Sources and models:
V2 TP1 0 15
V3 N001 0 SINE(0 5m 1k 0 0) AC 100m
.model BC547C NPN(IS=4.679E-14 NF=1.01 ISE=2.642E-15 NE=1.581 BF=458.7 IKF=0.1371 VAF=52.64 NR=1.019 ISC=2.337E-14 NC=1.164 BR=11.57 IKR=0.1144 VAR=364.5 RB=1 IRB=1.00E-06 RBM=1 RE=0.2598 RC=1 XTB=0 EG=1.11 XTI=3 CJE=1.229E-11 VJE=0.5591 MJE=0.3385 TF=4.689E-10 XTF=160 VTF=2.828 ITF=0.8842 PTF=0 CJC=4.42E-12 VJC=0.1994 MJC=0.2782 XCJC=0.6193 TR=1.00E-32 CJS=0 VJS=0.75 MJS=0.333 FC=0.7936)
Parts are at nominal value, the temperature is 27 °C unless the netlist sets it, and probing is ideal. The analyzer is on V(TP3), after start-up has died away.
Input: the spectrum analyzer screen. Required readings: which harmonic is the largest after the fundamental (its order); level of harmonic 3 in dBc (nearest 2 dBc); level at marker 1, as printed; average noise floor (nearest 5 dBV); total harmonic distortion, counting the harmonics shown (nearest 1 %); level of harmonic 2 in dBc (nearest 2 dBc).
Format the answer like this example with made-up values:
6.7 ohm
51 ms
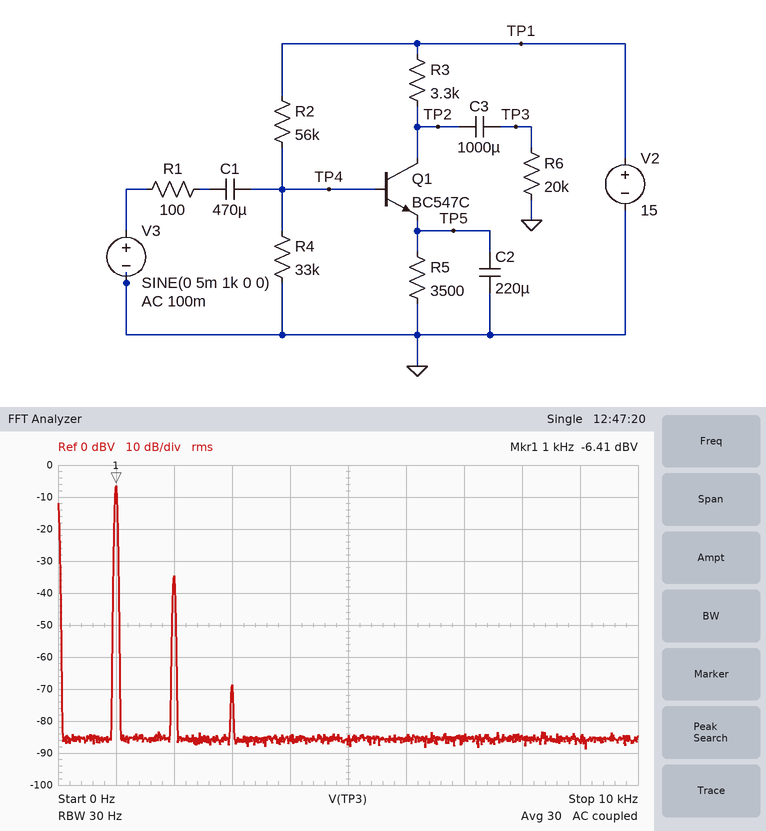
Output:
2
-62 dBc
-6.41 dBV
-85 dBV
4 %
-28 dBc
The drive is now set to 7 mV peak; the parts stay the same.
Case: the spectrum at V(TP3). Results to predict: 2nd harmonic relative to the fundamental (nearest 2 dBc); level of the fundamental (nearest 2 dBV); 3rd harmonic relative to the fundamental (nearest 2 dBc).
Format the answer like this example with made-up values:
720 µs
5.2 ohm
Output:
-26 dBc
-4 dBV
-56 dBc
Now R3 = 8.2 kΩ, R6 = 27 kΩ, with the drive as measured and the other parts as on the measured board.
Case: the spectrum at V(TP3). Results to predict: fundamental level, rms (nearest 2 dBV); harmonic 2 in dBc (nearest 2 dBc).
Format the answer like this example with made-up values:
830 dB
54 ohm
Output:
-32 dBV
-8 dBc
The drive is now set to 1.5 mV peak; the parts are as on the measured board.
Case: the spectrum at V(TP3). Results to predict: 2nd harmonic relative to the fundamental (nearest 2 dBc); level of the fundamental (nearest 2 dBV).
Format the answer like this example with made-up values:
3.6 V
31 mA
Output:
-38 dBc
-16 dBV
